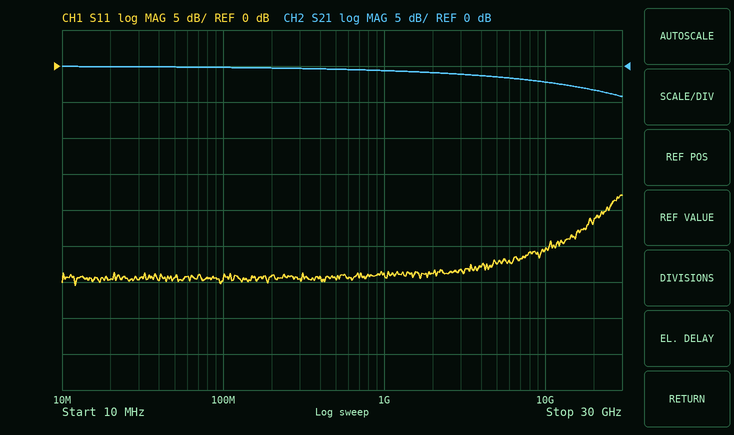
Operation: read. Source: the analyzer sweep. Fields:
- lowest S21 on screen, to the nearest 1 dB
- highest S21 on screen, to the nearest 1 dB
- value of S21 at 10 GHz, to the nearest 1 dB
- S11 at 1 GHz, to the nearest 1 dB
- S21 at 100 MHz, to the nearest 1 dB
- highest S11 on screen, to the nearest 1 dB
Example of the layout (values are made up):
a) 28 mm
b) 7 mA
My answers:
a) -4 dB
b) 0 dB
c) -2 dB
d) -29 dB
e) 0 dB
f) -18 dB
